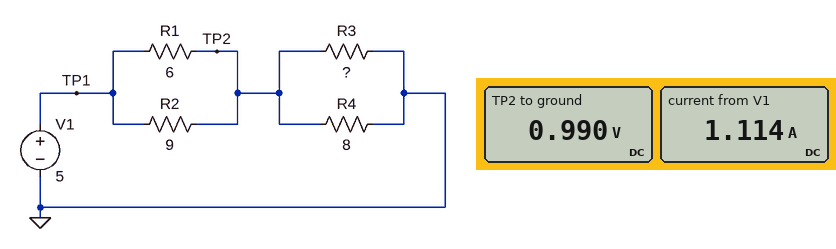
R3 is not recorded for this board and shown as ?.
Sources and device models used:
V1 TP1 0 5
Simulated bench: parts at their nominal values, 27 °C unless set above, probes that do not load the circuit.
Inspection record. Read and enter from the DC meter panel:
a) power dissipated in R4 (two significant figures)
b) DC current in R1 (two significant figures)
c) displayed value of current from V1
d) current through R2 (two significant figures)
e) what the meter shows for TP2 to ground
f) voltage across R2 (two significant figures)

120 mW
670 mA
1.114 A
450 mA
0.990 V
4.0 V
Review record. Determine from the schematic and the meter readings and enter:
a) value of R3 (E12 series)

1 Ω
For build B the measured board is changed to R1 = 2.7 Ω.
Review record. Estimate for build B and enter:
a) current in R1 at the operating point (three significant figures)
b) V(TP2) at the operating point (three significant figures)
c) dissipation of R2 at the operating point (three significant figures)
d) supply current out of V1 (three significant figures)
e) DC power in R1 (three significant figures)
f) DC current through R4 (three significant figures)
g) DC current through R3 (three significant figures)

1.30 A
1.50 V
1.36 W
1.69 A
4.54 W
187 mA
1.50 A
